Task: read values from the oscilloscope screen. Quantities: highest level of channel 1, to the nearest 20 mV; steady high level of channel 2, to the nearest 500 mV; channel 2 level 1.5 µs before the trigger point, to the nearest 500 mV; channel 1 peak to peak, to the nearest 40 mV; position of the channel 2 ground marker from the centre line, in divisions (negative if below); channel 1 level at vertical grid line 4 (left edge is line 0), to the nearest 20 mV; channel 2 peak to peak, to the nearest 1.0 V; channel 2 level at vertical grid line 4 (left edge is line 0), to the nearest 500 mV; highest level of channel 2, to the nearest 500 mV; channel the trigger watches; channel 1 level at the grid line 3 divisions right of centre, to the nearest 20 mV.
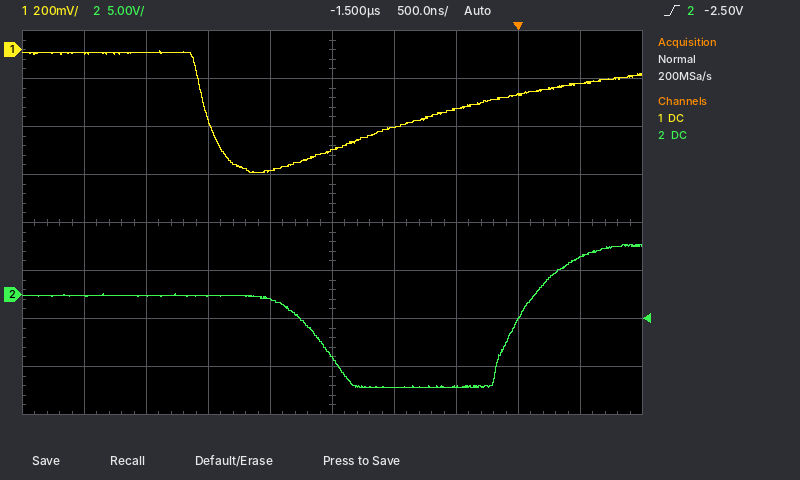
0 mV
0.0 V
-6.5 V
520 mV
-1.5 div
-500 mV
15.0 V
-500 mV
5.0 V
channel 2
-180 mV
